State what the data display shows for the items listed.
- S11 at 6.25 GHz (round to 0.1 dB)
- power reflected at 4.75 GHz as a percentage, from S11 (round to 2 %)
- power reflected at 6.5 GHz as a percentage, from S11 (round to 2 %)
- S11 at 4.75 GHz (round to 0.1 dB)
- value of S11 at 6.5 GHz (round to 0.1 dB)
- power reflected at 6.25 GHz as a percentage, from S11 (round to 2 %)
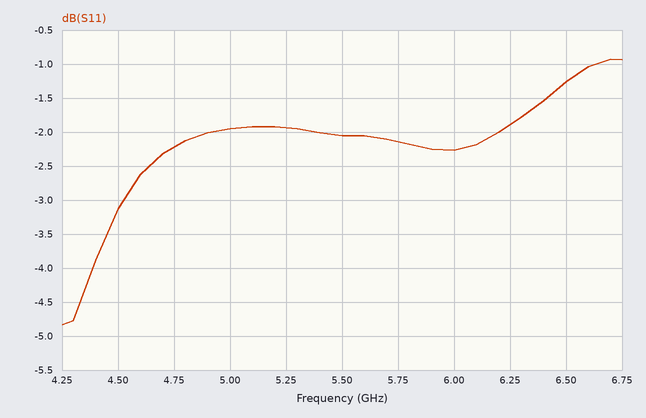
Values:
-1.9 dB
60 %
74 %
-2.2 dB
-1.3 dB
64 %
